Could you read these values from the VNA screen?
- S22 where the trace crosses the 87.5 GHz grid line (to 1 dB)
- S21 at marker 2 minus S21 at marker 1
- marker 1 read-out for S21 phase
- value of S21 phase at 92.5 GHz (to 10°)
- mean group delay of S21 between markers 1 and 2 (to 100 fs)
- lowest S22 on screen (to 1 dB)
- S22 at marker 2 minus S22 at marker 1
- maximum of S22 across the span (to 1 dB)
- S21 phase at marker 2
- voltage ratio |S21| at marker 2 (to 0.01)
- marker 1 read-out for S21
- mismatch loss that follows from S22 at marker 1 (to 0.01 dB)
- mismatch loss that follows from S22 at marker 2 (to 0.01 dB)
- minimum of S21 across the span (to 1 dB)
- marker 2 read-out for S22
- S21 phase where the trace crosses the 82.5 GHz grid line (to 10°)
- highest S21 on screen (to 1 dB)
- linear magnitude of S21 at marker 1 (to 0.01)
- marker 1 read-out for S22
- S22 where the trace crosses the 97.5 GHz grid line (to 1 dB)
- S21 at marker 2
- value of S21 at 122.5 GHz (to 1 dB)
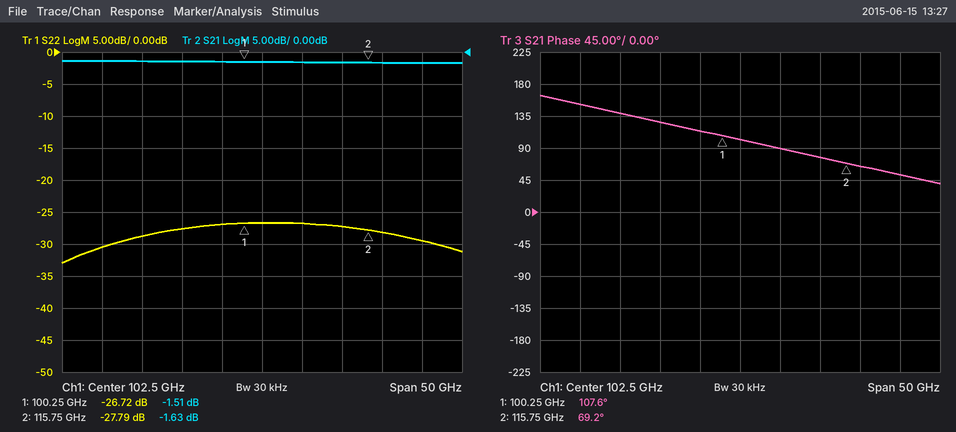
-29 dB
-0.12 dB
107.6°
130°
6.9 ps
-33 dB
-1.07 dB
-27 dB
69.2°
0.83
-1.51 dB
0.01 dB
0.01 dB
-2 dB
-27.79 dB
150°
-1 dB
0.84
-26.72 dB
-27 dB
-1.63 dB
-2 dB
